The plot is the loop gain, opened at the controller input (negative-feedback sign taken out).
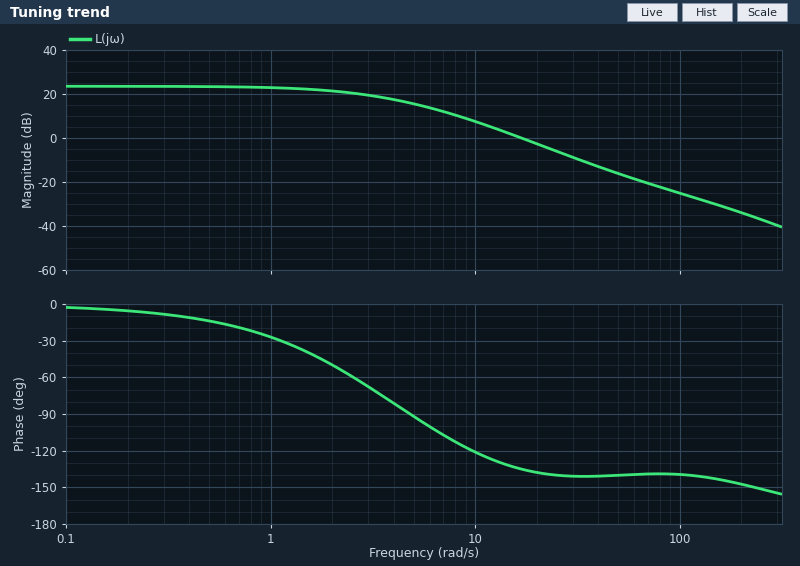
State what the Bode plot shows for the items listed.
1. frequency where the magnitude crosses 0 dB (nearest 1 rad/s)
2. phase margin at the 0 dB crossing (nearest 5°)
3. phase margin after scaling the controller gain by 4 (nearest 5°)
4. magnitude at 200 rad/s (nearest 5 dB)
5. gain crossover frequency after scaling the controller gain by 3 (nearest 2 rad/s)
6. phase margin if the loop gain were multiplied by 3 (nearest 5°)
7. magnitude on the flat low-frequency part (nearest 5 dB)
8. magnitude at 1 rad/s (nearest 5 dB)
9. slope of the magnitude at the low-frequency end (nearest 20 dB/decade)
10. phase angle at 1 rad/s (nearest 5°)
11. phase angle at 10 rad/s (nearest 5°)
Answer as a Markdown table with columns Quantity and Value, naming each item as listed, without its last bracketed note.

| Quantity | Value |
|---|---|
| frequency where the magnitude crosses 0 dB | 17 rad/s |
| phase margin at the 0 dB crossing | 45° |
| phase margin after scaling the controller gain by 4 | 40° |
| magnitude at 200 rad/s | -35 dB |
| gain crossover frequency after scaling the controller gain by 3 | 32 rad/s |
| phase margin if the loop gain were multiplied by 3 | 40° |
| magnitude on the flat low-frequency part | 25 dB |
| magnitude at 1 rad/s | 25 dB |
| slope of the magnitude at the low-frequency end | 0 dB/decade |
| phase angle at 1 rad/s | -25° |
| phase angle at 10 rad/s | -120° |
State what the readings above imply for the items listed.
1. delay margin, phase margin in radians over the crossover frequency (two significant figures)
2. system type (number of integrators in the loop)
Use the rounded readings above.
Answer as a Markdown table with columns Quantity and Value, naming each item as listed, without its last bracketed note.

| Quantity | Value |
|---|---|
| delay margin, phase margin in radians over the crossover frequency | 0.046 s |
| system type | 0 |
